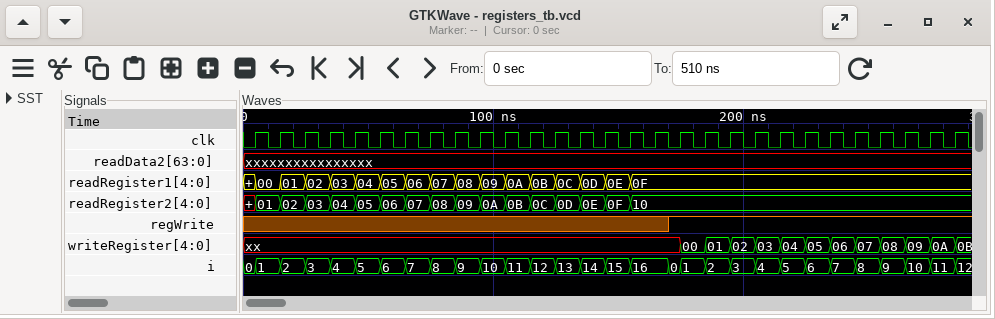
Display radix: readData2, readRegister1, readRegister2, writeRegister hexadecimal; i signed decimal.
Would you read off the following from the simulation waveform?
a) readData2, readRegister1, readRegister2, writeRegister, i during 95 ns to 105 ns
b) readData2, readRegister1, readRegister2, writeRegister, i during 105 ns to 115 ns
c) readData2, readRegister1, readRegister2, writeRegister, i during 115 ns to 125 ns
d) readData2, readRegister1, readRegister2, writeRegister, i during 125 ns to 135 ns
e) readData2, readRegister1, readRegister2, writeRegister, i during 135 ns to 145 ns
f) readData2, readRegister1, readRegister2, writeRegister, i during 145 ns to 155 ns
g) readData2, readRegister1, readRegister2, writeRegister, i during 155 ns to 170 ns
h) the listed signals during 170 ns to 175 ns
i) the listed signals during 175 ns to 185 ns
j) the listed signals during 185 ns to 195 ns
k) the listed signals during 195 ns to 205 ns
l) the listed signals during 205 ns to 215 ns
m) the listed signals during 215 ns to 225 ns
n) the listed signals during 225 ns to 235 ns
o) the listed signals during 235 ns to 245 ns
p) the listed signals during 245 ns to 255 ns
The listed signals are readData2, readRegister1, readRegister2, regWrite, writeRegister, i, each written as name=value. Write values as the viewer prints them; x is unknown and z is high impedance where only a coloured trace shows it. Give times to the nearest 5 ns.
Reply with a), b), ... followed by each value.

a) readData2=xxxxxxxxxxxxxxxx, readRegister1=09, readRegister2=0A, writeRegister=xx, i=10
b) readData2=xxxxxxxxxxxxxxxx, readRegister1=0A, readRegister2=0B, writeRegister=xx, i=11
c) readData2=xxxxxxxxxxxxxxxx, readRegister1=0B, readRegister2=0C, writeRegister=xx, i=12
d) readData2=xxxxxxxxxxxxxxxx, readRegister1=0C, readRegister2=0D, writeRegister=xx, i=13
e) readData2=xxxxxxxxxxxxxxxx, readRegister1=0D, readRegister2=0E, writeRegister=xx, i=14
f) readData2=xxxxxxxxxxxxxxxx, readRegister1=0E, readRegister2=0F, writeRegister=xx, i=15
g) readData2=xxxxxxxxxxxxxxxx, readRegister1=0F, readRegister2=10, writeRegister=xx, i=16
h) readData2=xxxxxxxxxxxxxxxx, readRegister1=0F, readRegister2=10, regWrite=1, writeRegister=xx, i=0
i) readData2=xxxxxxxxxxxxxxxx, readRegister1=0F, readRegister2=10, regWrite=1, writeRegister=00, i=1
j) readData2=xxxxxxxxxxxxxxxx, readRegister1=0F, readRegister2=10, regWrite=1, writeRegister=01, i=2
k) readData2=xxxxxxxxxxxxxxxx, readRegister1=0F, readRegister2=10, regWrite=1, writeRegister=02, i=3
l) readData2=xxxxxxxxxxxxxxxx, readRegister1=0F, readRegister2=10, regWrite=1, writeRegister=03, i=4
m) readData2=xxxxxxxxxxxxxxxx, readRegister1=0F, readRegister2=10, regWrite=1, writeRegister=04, i=5
n) readData2=xxxxxxxxxxxxxxxx, readRegister1=0F, readRegister2=10, regWrite=1, writeRegister=05, i=6
o) readData2=xxxxxxxxxxxxxxxx, readRegister1=0F, readRegister2=10, regWrite=1, writeRegister=06, i=7
p) readData2=xxxxxxxxxxxxxxxx, readRegister1=0F, readRegister2=10, regWrite=1, writeRegister=07, i=8
